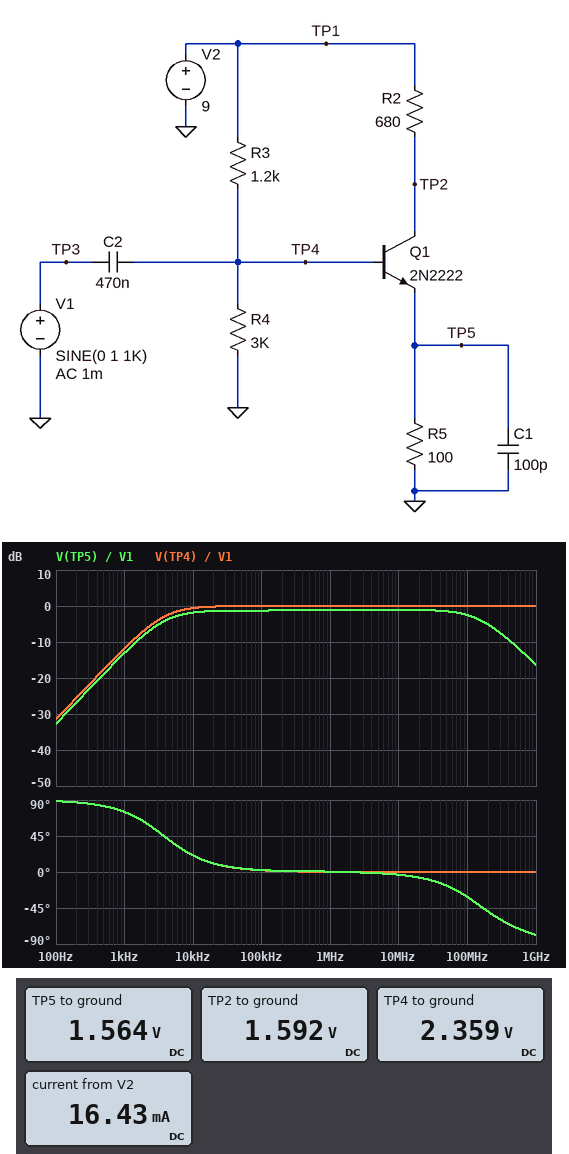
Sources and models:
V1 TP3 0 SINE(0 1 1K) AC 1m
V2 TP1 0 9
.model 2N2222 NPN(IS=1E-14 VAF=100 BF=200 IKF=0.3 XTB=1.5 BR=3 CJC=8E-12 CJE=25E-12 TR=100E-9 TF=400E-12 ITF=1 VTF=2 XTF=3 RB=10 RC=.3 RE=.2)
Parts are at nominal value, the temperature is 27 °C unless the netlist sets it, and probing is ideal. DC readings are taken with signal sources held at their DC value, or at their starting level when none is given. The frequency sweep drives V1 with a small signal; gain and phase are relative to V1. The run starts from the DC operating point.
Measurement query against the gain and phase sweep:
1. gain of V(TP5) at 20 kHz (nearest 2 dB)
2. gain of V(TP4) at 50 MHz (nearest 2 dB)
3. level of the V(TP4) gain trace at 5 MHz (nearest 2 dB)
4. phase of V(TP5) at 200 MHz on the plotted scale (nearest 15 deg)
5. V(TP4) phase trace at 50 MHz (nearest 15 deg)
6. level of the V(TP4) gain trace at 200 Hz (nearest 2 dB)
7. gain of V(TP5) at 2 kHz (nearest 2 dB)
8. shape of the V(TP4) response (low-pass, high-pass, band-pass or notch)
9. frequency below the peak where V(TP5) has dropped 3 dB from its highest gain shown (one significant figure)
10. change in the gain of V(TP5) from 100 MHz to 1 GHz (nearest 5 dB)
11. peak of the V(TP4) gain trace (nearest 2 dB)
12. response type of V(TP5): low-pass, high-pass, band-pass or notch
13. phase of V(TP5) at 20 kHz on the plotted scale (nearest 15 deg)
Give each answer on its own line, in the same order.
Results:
-2 dB
0 dB
0 dB
-45 deg
0 deg
-26 dB
-8 dB
high-pass
4 kHz
-15 dB
0 dB
band-pass
15 deg
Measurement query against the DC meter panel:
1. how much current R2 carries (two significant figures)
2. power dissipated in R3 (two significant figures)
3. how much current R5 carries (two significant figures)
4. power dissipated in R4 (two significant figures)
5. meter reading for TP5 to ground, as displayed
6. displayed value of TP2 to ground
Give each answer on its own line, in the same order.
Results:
11 mA
37 mW
16 mA
1.9 mW
1.564 V
1.592 V
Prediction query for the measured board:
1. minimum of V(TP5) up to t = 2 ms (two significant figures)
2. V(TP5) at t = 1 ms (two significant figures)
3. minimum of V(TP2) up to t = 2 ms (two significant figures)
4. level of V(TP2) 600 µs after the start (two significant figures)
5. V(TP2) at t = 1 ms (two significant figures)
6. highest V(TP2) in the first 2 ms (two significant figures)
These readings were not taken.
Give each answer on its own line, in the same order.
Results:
1.3 V
1.8 V
1.4 V
1.4 V
1.8 V
1.8 V
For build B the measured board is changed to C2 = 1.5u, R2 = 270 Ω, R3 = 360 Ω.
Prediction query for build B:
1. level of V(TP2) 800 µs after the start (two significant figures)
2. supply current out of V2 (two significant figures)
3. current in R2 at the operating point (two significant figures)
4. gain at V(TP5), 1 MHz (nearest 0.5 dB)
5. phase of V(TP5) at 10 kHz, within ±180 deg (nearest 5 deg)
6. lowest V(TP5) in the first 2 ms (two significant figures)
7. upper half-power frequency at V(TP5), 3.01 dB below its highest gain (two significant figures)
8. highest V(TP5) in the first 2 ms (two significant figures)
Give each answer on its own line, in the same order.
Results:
3.2 V
34 mA
21 mA
-1.0 dB
10 deg
2.8 V
170 MHz
3.8 V
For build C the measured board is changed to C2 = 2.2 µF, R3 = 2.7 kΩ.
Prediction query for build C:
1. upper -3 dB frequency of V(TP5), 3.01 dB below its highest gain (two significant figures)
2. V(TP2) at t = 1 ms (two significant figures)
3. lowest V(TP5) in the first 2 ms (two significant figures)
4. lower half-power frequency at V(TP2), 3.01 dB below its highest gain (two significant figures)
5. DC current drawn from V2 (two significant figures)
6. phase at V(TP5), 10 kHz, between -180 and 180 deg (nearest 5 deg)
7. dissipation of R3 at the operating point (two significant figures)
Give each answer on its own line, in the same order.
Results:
150 MHz
1.3 V
99 mV
1.1 kHz
14 mA
5 deg
18 mW
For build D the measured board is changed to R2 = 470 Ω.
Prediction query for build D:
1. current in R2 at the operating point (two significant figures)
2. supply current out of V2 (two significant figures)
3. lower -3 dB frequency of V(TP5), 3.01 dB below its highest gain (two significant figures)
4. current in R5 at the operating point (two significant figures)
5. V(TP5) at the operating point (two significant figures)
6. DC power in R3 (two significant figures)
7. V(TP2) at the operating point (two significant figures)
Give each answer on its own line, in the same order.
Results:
15 mA
20 mA
4.1 kHz
19 mA
1.9 V
33 mW
2.0 V
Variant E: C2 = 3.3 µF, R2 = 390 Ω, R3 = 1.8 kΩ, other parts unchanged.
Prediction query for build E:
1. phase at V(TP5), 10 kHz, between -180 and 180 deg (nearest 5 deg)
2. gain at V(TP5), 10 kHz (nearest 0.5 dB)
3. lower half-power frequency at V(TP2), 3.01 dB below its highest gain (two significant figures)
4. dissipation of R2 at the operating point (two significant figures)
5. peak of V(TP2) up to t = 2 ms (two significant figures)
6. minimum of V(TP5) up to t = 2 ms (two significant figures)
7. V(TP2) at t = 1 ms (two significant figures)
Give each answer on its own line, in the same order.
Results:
5 deg
-1.5 dB
740 Hz
120 mW
5.9 V
800 mV
2.0 V
